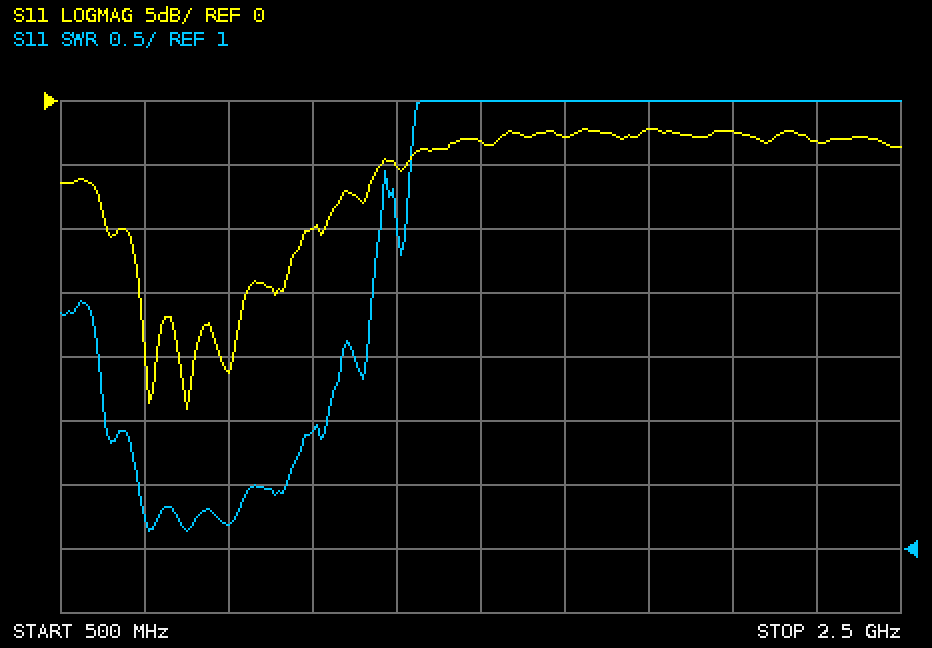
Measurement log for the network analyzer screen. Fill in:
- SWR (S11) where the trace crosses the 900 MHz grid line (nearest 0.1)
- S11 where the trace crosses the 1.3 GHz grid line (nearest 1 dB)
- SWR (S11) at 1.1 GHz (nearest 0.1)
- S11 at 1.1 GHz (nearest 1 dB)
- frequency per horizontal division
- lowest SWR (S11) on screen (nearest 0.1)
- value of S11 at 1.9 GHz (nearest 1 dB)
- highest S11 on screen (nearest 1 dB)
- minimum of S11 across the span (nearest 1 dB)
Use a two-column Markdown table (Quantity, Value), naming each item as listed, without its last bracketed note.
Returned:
| Quantity | Value |
|---|---|
| SWR (S11) where the trace crosses the 900 MHz grid line | 1.2 |
| S11 where the trace crosses the 1.3 GHz grid line | -5 dB |
| SWR (S11) at 1.1 GHz | 1.9 |
| S11 at 1.1 GHz | -10 dB |
| frequency per horizontal division | 200 MHz |
| lowest SWR (S11) on screen | 1.1 |
| value of S11 at 1.9 GHz | -2 dB |
| highest S11 on screen | -2 dB |
| minimum of S11 across the span | -24 dB |
